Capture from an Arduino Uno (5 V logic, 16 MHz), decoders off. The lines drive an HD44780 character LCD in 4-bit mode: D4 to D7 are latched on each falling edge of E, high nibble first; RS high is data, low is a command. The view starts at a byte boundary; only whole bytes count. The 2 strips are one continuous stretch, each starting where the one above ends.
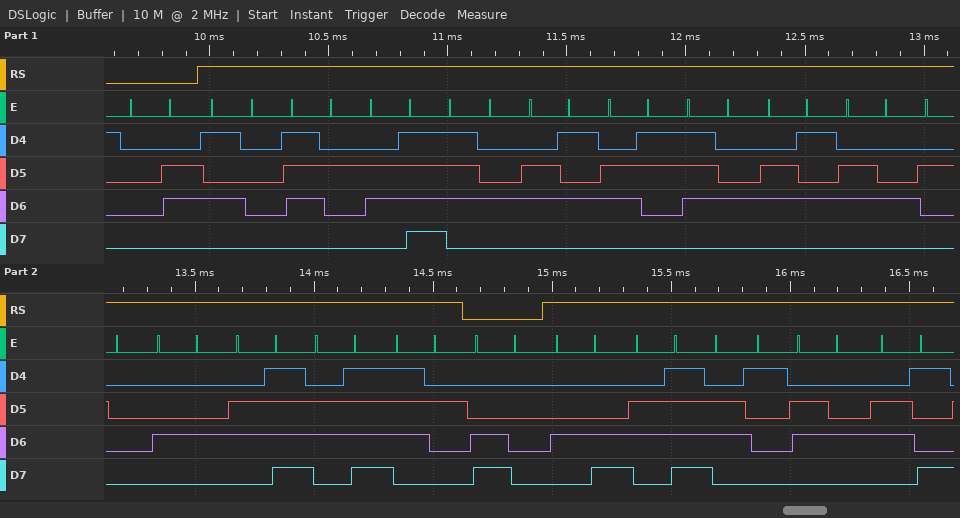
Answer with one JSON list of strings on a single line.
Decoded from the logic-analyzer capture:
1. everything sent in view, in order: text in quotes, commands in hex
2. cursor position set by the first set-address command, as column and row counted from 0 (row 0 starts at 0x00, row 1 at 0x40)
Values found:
["0x06 \"Protected Door\" 0xC0 \"Loadi\"", "column 0, row 1"]
